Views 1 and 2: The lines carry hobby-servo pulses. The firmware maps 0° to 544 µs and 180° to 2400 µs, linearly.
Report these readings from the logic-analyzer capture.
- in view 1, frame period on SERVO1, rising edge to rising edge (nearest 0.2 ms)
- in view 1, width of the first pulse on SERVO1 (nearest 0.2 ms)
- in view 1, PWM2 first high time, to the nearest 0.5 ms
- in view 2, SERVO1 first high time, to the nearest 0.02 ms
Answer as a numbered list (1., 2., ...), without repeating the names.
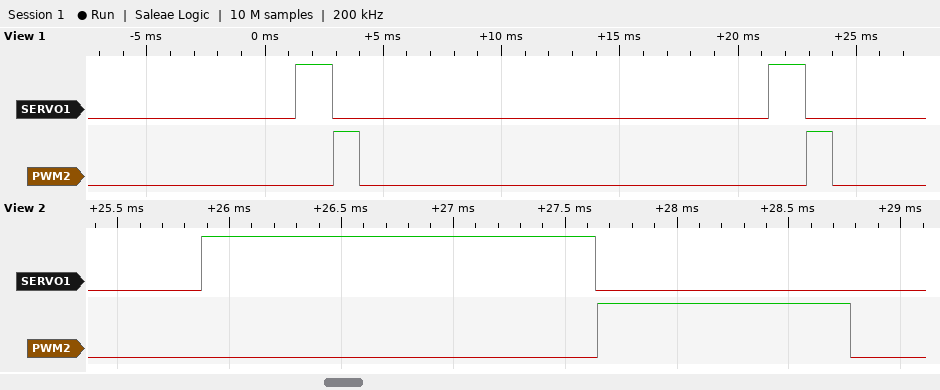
1. 20.0 ms
2. 1.6 ms
3. 1.0 ms
4. 1.76 ms
